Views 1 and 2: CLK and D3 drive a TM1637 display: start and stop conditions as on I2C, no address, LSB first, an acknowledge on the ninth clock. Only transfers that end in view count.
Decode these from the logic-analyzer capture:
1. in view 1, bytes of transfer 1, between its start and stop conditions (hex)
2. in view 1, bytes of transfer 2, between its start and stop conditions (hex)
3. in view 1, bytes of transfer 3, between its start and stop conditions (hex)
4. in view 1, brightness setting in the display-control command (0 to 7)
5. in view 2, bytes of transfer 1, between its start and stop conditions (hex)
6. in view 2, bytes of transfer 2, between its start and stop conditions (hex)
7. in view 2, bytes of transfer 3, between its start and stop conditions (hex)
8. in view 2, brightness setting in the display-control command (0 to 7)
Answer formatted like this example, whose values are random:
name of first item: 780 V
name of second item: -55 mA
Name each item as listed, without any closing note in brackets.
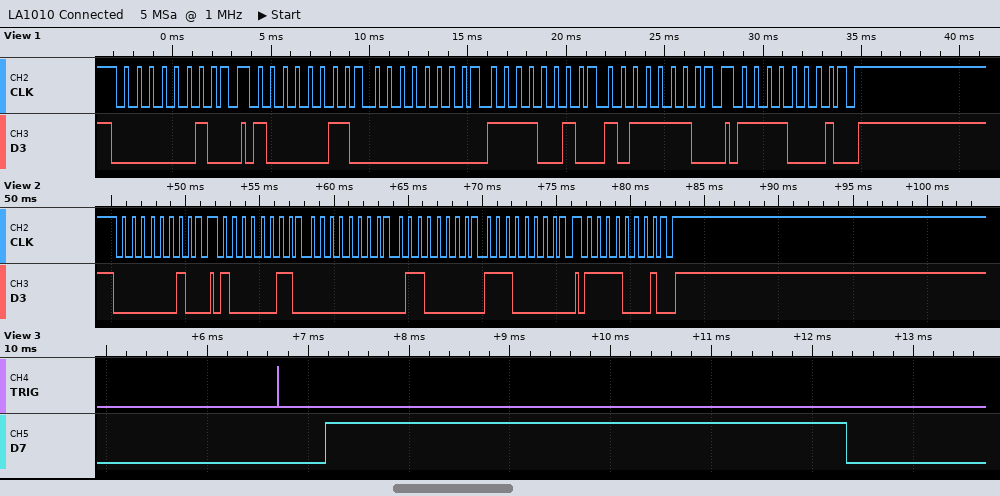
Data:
in view 1, bytes of transfer 1, between its start and stop conditions: 40
in view 1, bytes of transfer 2, between its start and stop conditions: C1 00 4F 7D
in view 1, bytes of transfer 3, between its start and stop conditions: 8F
in view 1, brightness setting in the display-control command: 7
in view 2, bytes of transfer 1, between its start and stop conditions: 40
in view 2, bytes of transfer 2, between its start and stop conditions: C1 00 06 07
in view 2, bytes of transfer 3, between its start and stop conditions: 8F
in view 2, brightness setting in the display-control command: 7
